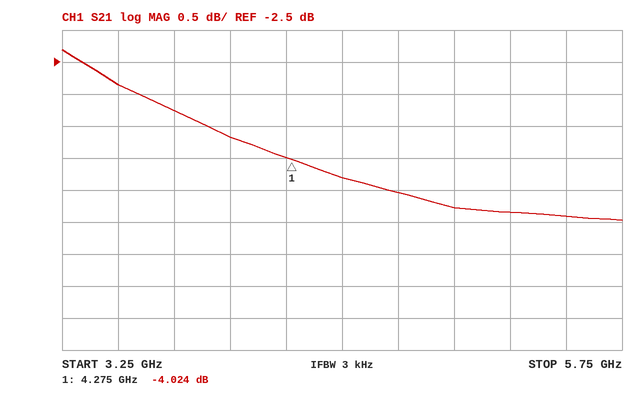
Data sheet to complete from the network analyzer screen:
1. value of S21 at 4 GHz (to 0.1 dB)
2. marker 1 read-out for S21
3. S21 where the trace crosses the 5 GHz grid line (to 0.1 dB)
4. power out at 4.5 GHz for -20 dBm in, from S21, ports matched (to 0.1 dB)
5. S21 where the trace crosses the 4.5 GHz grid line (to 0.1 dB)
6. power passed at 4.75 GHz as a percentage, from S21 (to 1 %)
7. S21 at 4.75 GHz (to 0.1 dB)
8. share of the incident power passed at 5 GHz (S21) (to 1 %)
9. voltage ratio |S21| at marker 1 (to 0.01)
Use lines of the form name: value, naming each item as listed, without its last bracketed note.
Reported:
value of S21 at 4 GHz: -3.7 dB
marker 1 read-out for S21: -4.024 dB
S21 where the trace crosses the 5 GHz grid line: -4.8 dB
power out at 4.5 GHz for -20 dBm in, from S21, ports matched: -24.3 dBm
S21 where the trace crosses the 4.5 GHz grid line: -4.3 dB
power passed at 4.75 GHz as a percentage, from S21: 35 %
S21 at 4.75 GHz: -4.5 dB
share of the incident power passed at 5 GHz (S21): 33 %
voltage ratio |S21| at marker 1: 0.63
